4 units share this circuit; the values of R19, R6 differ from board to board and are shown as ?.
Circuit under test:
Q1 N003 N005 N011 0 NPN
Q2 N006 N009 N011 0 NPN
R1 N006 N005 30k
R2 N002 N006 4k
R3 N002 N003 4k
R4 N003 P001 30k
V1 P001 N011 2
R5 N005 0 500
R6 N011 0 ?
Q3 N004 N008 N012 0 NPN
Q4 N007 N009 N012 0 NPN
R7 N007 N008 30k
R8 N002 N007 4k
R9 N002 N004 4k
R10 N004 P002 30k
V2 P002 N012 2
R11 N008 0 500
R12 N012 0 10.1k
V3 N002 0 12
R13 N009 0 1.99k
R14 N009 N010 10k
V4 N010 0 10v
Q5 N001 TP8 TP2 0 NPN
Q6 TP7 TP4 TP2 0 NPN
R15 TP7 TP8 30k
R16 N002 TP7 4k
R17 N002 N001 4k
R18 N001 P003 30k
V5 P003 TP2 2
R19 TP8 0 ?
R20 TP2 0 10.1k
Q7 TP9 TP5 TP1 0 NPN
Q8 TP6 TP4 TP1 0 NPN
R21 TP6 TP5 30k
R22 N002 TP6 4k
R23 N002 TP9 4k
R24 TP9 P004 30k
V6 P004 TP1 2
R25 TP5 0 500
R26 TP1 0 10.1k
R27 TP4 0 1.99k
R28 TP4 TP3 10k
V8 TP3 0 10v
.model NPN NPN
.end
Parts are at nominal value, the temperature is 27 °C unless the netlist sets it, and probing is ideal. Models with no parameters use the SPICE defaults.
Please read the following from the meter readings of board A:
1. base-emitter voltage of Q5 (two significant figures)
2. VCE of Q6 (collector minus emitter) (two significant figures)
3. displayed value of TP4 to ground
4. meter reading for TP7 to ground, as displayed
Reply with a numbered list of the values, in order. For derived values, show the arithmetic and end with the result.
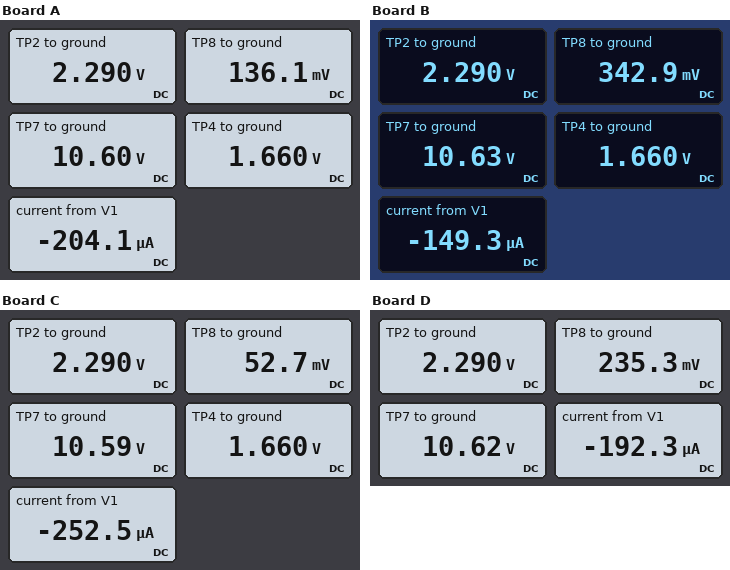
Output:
1. 136.1 mV - 2.29 V = -2.2 V
2. 10.6 V - 2.29 V = 8.3 V
3. 1.660 V
4. 10.60 V
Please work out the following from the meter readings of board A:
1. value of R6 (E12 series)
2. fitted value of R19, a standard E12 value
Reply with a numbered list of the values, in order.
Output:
1. 15 kΩ
2. 390 Ω
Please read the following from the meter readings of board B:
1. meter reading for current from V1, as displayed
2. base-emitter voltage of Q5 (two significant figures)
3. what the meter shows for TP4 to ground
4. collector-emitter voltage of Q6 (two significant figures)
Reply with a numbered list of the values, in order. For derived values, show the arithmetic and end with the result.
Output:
1. -149.3 µA
2. 342.9 mV - 2.29 V = -1.9 V
3. 1.660 V
4. 10.63 V - 2.29 V = 8.3 V
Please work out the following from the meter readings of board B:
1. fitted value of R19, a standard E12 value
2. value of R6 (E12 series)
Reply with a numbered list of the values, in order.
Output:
1. 1 kΩ
2. 33 kΩ
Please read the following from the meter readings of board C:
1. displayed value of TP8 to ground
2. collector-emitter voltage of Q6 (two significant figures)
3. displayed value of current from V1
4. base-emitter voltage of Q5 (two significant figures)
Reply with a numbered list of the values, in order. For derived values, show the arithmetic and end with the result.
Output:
1. 52.7 mV
2. 10.59 V - 2.29 V = 8.3 V
3. -252.5 µA
4. 52.7 mV - 2.29 V = -2.2 V
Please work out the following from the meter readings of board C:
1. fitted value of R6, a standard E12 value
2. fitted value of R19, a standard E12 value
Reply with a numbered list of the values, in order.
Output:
1. 5.6 kΩ
2. 150 Ω
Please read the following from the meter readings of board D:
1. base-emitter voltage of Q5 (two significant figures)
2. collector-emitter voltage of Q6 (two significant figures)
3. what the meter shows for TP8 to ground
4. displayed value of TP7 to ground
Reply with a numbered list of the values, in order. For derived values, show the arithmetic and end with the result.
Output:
1. 235.3 mV - 2.29 V = -2.1 V
2. 10.62 V - 2.29 V = 8.3 V
3. 235.3 mV
4. 10.62 V
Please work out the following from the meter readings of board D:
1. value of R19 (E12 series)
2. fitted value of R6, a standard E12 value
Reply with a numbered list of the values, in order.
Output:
1. 680 Ω
2. 18 kΩ
